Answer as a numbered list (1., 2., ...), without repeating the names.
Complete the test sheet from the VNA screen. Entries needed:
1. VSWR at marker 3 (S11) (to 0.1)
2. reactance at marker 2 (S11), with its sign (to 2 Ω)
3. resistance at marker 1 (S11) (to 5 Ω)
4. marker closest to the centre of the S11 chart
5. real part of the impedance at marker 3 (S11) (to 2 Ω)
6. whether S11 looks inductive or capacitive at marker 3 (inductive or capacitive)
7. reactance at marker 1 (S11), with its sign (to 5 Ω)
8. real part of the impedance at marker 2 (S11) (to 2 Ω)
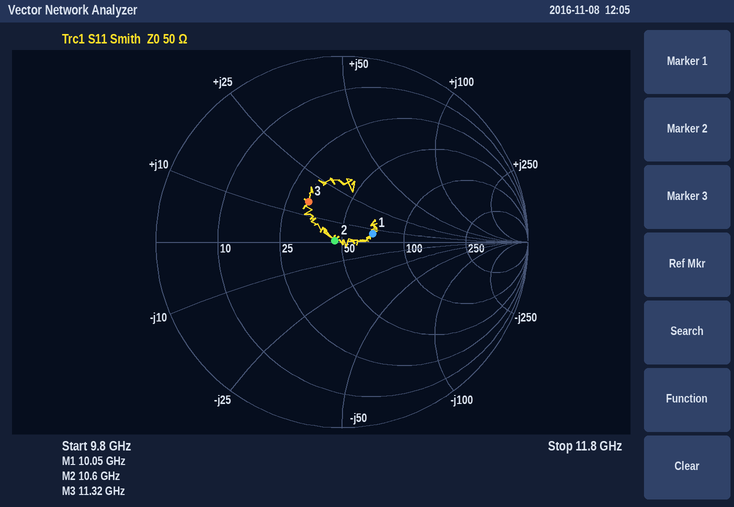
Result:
1. 1.8
2. 0 Ω
3. 70 Ω
4. marker 2
5. 32 Ω
6. inductive
7. +5 Ω
8. 46 Ω
